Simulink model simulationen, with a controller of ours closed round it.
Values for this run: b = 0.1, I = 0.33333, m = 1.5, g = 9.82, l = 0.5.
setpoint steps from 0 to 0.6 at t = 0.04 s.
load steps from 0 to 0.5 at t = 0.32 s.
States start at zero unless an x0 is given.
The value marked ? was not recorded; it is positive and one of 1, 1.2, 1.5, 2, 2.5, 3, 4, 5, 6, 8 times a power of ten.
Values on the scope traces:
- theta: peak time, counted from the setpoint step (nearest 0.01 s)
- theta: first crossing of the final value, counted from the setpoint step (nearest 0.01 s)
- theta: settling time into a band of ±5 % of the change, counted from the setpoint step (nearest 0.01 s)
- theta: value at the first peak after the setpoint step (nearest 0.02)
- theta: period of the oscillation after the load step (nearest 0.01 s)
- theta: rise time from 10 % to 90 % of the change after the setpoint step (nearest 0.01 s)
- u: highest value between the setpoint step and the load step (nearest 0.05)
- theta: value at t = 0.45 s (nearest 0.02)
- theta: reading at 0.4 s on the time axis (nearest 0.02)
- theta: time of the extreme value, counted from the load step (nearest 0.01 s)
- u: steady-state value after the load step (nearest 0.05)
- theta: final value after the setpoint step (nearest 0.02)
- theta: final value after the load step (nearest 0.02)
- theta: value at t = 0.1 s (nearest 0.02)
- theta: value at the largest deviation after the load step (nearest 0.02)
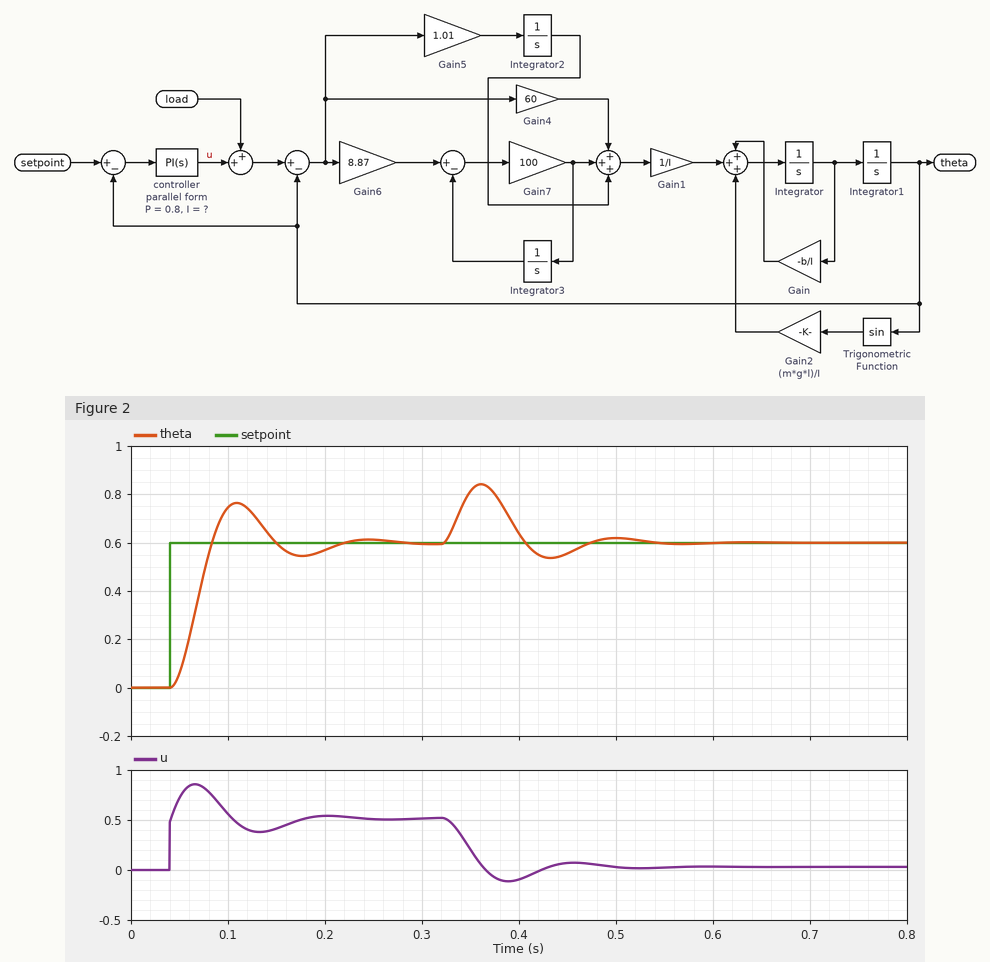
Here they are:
0.07 s
0.04 s
0.16 s
0.76
0.14 s
0.03 s
0.85
0.56
0.64
0.04 s
0.05
0.60
0.60
0.74
0.84
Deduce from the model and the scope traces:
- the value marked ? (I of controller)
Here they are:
50
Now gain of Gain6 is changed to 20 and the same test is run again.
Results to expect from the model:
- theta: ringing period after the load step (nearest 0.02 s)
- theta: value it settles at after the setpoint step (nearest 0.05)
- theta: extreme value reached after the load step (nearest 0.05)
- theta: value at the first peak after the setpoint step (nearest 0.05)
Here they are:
0.08 s
0.60
0.90
0.65
